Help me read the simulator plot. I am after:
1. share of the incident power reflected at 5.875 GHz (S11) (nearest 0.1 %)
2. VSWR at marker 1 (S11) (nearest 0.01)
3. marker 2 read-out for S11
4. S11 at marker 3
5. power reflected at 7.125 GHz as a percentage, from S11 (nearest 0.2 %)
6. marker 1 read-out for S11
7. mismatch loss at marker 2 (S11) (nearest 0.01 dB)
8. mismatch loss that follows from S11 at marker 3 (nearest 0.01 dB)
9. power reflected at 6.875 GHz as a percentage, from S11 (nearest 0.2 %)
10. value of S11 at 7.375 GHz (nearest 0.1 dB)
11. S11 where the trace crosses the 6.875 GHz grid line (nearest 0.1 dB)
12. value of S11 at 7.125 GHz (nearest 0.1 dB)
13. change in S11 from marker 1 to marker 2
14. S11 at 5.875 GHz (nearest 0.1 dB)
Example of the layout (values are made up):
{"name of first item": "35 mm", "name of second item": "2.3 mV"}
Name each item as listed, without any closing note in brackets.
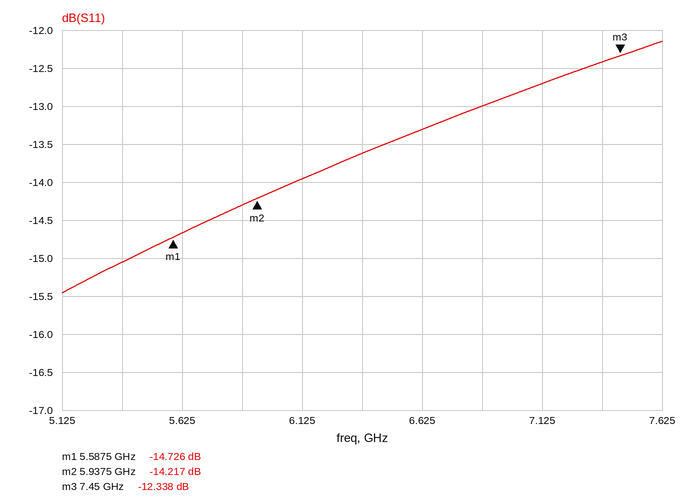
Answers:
{"share of the incident power reflected at 5.875 GHz (S11)": "3.7 %", "VSWR at marker 1 (S11)": "1.45", "marker 2 read-out for S11": "-14.217 dB", "S11 at marker 3": "-12.338 dB", "power reflected at 7.125 GHz as a percentage, from S11": "5.4 %", "marker 1 read-out for S11": "-14.726 dB", "mismatch loss at marker 2 (S11)": "0.17 dB", "mismatch loss that follows from S11 at marker 3": "0.26 dB", "power reflected at 6.875 GHz as a percentage, from S11": "5.0 %", "value of S11 at 7.375 GHz": "-12.4 dB", "S11 where the trace crosses the 6.875 GHz grid line": "-13.0 dB", "value of S11 at 7.125 GHz": "-12.7 dB", "change in S11 from marker 1 to marker 2": "0.509 dB", "S11 at 5.875 GHz": "-14.3 dB"}
